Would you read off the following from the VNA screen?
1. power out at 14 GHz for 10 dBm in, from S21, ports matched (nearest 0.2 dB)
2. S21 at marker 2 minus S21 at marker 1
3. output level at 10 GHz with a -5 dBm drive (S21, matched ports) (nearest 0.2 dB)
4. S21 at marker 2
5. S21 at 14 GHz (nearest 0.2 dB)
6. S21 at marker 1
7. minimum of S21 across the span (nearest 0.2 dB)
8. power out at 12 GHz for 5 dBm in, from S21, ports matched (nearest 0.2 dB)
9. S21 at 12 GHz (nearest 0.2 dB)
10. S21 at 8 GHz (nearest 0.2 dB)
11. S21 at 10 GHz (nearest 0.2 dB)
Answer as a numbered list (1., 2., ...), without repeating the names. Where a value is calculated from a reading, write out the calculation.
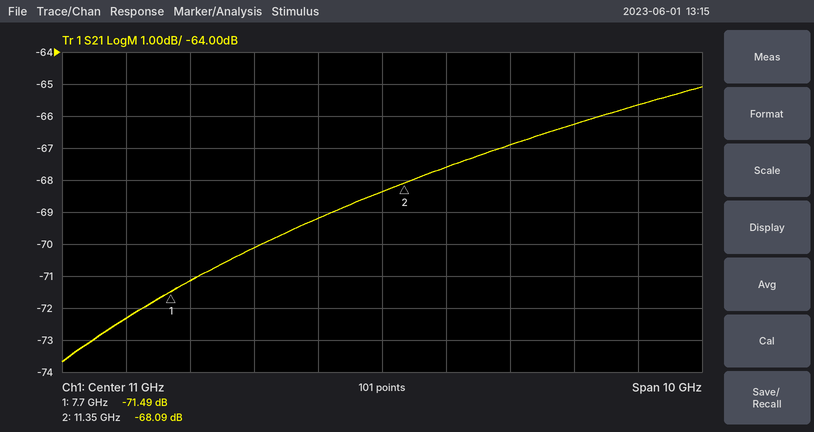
1. 10 dBm + (-66.2 dB) = -56.2 dBm
2. -68.09 − (-71.49) = 3.40 dB
3. -5 dBm + (-69.2 dB) = -74.2 dBm
4. -68.09 dB
5. -66.2 dB
6. -71.49 dB
7. -73.6 dB
8. 5 dBm + (-67.6 dB) = -62.6 dBm
9. -67.6 dB
10. -71.2 dB
11. -69.2 dB
